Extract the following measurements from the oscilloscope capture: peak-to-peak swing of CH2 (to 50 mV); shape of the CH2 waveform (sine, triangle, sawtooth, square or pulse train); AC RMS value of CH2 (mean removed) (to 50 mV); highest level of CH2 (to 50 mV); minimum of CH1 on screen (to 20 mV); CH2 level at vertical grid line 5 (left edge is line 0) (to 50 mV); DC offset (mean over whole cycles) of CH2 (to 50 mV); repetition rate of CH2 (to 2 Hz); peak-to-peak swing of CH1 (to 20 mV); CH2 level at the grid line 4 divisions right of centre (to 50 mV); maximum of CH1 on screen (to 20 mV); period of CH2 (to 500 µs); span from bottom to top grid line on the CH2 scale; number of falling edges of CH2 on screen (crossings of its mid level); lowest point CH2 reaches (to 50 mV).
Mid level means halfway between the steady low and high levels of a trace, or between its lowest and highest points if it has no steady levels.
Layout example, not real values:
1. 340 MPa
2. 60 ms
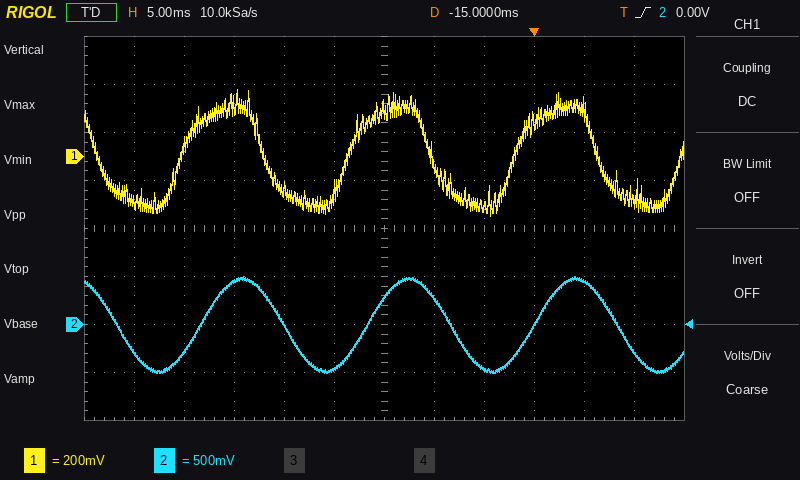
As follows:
1. 1.00 V
2. sine
3. 350 mV
4. 500 mV
5. -240 mV
6. -450 mV
7. 0 mV
8. 60 Hz
9. 520 mV
10. 450 mV
11. 280 mV
12. 16.5 ms
13. 4 V
14. 4
15. -500 mV
